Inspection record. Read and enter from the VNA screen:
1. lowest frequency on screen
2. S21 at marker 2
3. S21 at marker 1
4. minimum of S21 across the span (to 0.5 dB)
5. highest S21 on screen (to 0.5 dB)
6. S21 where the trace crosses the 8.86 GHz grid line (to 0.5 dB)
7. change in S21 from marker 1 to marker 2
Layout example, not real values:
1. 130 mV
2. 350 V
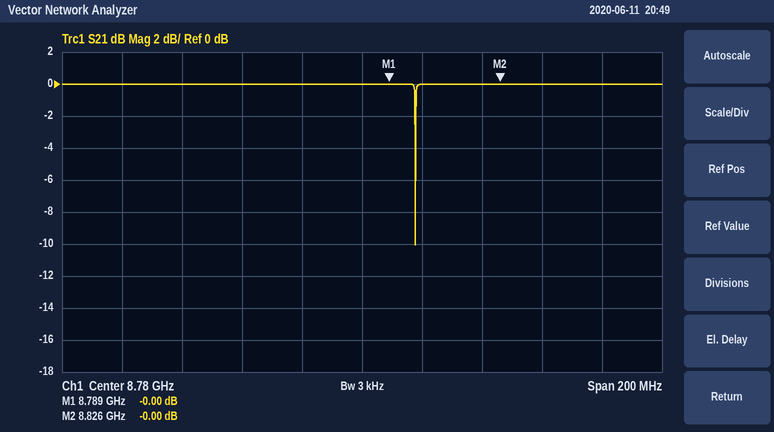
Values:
1. 8.68 GHz
2. -0.00 dB
3. -0.00 dB
4. -10.0 dB
5. 0.0 dB
6. 0.0 dB
7. 0.00 dB
